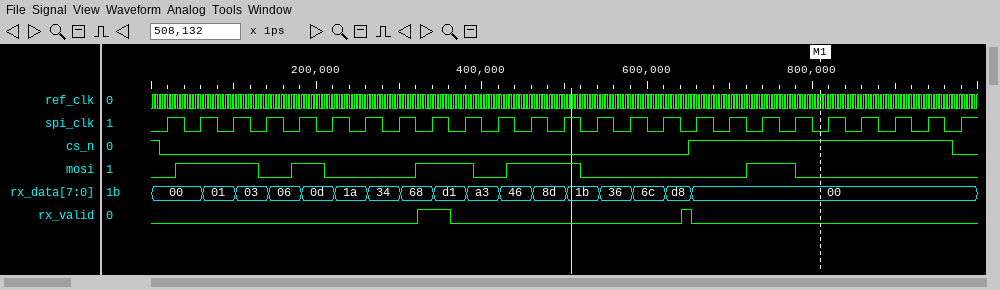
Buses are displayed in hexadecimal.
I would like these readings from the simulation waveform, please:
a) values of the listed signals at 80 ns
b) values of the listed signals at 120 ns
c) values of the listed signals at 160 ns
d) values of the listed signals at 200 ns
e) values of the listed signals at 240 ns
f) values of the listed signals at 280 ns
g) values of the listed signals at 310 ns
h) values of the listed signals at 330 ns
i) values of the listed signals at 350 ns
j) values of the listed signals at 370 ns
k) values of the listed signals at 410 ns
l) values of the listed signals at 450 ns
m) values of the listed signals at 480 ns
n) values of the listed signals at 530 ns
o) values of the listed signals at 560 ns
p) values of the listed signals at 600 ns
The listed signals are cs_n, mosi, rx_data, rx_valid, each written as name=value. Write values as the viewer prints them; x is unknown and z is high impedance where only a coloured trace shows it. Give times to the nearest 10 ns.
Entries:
cs_n=0, mosi=1, rx_data=01, rx_valid=0
cs_n=0, mosi=1, rx_data=03, rx_valid=0
cs_n=0, mosi=0, rx_data=06, rx_valid=0
cs_n=0, mosi=1, rx_data=0d, rx_valid=0
cs_n=0, mosi=0, rx_data=1a, rx_valid=0
cs_n=0, mosi=0, rx_data=34, rx_valid=0
cs_n=0, mosi=0, rx_data=68, rx_valid=0
cs_n=0, mosi=1, rx_data=68, rx_valid=1
cs_n=0, mosi=1, rx_data=d1, rx_valid=1
cs_n=0, mosi=1, rx_data=d1, rx_valid=0
cs_n=0, mosi=0, rx_data=a3, rx_valid=0
cs_n=0, mosi=1, rx_data=46, rx_valid=0
cs_n=0, mosi=1, rx_data=8d, rx_valid=0
cs_n=0, mosi=0, rx_data=1b, rx_valid=0
cs_n=0, mosi=0, rx_data=36, rx_valid=0
cs_n=0, mosi=0, rx_data=6c, rx_valid=0
